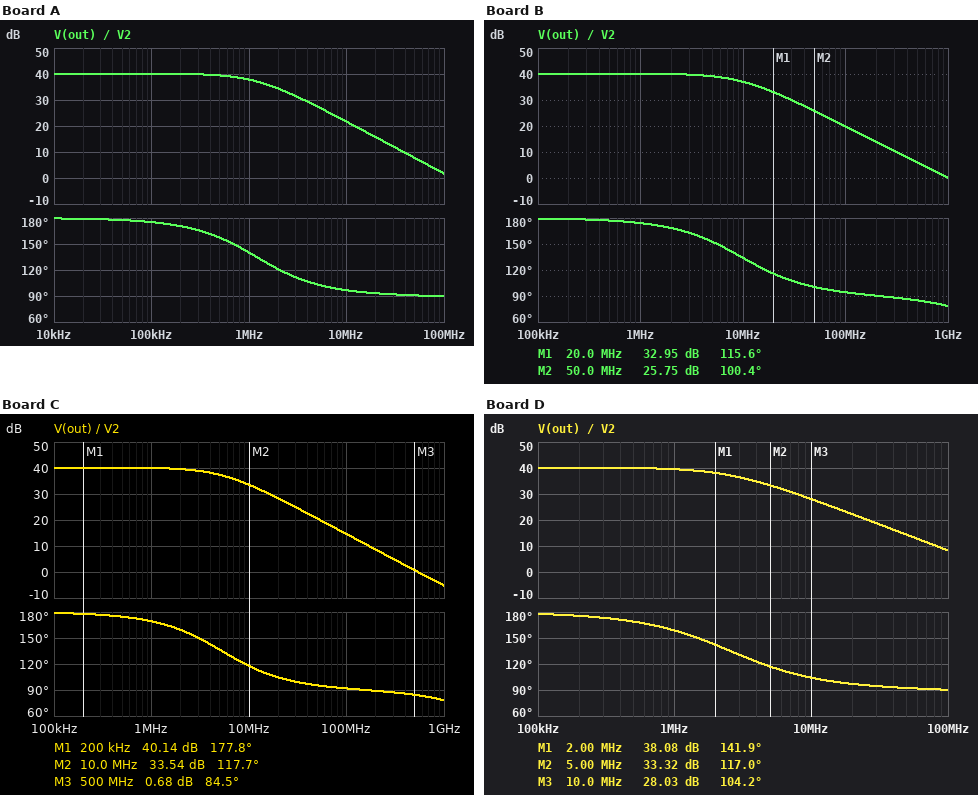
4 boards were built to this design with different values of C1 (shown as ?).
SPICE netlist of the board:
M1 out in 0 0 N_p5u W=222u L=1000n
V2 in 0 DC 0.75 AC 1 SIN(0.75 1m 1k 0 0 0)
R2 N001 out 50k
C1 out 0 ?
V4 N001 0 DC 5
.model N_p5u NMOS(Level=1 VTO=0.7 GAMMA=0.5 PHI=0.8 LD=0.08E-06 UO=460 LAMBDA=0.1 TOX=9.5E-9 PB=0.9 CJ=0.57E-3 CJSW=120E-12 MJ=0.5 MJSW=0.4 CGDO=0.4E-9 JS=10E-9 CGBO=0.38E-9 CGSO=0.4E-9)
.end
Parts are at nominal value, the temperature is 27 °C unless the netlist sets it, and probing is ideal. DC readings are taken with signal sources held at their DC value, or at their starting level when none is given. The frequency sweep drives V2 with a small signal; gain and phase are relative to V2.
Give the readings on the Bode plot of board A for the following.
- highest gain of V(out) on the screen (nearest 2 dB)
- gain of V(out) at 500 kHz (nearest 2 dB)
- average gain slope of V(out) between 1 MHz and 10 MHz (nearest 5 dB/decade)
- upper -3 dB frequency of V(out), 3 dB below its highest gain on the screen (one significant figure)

40 dB
40 dB
-15 dB/decade
1 MHz
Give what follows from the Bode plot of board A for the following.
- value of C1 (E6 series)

3.3 pF
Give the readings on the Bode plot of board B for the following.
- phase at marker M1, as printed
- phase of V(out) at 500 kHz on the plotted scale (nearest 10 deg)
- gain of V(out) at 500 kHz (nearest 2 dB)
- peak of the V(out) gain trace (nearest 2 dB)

115.6 deg
180 deg
40 dB
40 dB
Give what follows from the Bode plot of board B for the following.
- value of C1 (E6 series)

330 fF
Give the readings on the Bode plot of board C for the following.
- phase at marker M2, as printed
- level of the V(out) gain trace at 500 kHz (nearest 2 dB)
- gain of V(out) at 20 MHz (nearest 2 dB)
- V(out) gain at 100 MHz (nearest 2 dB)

117.7 deg
40 dB
28 dB
14 dB
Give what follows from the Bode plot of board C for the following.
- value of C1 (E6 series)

680 fF
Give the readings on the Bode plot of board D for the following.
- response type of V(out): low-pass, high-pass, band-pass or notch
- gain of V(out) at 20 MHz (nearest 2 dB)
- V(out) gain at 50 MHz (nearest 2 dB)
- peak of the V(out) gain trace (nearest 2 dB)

low-pass
22 dB
14 dB
40 dB
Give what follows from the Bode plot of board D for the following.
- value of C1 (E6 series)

1.5 pF
